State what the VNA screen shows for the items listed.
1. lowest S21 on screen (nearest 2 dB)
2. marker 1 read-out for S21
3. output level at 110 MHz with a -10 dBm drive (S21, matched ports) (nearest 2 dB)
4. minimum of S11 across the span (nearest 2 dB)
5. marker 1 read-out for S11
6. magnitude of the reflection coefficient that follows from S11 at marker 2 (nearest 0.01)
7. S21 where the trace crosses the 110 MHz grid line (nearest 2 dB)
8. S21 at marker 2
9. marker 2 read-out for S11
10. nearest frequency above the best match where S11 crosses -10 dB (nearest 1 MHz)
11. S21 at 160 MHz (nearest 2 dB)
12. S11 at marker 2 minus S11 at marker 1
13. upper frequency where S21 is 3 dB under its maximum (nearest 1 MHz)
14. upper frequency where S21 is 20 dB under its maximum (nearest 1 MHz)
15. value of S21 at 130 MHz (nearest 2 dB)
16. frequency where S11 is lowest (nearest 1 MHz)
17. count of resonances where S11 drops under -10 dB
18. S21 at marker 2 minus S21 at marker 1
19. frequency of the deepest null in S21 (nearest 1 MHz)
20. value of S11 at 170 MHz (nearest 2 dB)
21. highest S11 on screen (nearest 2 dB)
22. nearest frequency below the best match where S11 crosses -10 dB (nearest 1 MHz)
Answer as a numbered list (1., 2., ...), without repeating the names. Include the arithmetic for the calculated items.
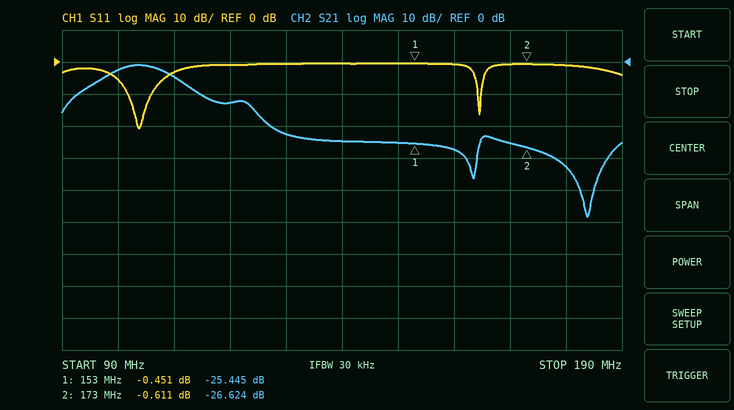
1. -48 dB
2. -25.445 dB
3. -10 dBm + (-4 dB) = -14 dBm
4. -20 dB
5. -0.451 dB
6. 10^(-0.611/20) ≈ 0.93
7. -4 dB
8. -26.624 dB
9. -0.611 dB
10. 106 MHz
11. -28 dB
12. -0.611 − (-0.451) = -0.160 dB
13. 109 MHz
14. 128 MHz
15. -22 dB
16. 104 MHz
17. 2
18. -26.624 − (-25.445) = -1.179 dB
19. 184 MHz
20. 0 dB
21. 0 dB
22. 102 MHz
